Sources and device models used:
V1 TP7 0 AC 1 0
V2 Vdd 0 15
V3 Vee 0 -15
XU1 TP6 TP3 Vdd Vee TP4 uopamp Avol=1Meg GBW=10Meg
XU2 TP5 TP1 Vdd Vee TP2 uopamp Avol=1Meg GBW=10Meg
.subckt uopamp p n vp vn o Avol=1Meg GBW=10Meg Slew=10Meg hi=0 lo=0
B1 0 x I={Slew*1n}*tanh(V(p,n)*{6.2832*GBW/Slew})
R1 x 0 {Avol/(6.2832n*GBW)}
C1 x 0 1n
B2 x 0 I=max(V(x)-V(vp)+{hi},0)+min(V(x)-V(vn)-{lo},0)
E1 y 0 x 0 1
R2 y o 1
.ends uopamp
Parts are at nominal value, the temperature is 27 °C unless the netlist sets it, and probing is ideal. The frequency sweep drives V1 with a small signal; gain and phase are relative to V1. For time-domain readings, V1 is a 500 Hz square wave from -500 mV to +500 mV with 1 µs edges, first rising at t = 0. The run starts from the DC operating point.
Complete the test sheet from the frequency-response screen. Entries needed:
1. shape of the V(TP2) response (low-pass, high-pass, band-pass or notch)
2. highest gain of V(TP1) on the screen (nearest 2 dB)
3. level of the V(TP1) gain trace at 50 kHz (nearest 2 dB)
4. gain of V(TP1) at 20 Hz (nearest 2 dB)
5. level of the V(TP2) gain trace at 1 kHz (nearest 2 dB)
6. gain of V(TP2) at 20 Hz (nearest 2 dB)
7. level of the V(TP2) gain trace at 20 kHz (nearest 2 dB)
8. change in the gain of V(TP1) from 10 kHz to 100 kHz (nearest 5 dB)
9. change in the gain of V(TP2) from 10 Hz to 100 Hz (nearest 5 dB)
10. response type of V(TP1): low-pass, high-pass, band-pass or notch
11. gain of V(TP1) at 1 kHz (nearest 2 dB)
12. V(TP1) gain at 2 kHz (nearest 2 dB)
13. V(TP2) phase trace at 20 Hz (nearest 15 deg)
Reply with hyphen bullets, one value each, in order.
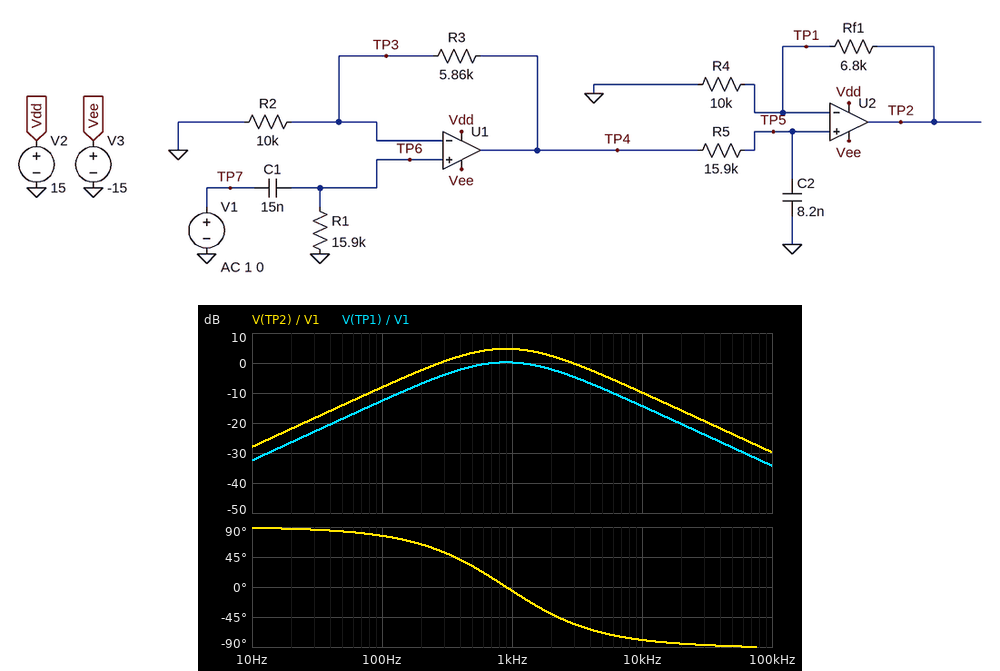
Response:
- band-pass
- 0 dB
- -28 dB
- -26 dB
- 4 dB
- -22 dB
- -16 dB
- -20 dB
- 20 dB
- band-pass
- 0 dB
- -2 dB
- 90 deg
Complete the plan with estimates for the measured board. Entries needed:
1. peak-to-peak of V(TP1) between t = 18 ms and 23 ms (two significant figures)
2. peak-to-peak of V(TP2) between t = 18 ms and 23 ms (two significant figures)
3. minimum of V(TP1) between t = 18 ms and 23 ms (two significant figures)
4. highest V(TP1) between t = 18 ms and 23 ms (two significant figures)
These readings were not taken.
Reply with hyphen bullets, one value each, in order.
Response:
- 1.5 V
- 2.5 V
- -740 mV
- 740 mV
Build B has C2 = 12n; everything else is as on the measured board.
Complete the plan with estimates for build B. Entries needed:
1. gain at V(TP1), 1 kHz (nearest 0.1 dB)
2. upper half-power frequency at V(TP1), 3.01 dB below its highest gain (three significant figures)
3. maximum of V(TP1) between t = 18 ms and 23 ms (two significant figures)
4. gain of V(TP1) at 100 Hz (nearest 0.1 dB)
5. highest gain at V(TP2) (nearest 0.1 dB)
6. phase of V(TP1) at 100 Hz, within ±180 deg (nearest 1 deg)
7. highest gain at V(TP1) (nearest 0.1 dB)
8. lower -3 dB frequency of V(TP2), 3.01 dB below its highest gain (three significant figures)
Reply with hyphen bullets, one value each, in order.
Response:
- -1.5 dB
- 1.81 kHz
- 620 mV
- -12.6 dB
- 3.4 dB
- 75 deg
- -1.1 dB
- 308 Hz
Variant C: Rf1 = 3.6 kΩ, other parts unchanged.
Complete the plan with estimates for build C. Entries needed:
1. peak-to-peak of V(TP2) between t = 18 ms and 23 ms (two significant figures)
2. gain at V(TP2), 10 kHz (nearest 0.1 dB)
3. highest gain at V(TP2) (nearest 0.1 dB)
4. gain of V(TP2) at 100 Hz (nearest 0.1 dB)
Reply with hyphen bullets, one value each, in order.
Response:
- 2.0 V
- -11.7 dB
- 2.9 dB
- -9.9 dB
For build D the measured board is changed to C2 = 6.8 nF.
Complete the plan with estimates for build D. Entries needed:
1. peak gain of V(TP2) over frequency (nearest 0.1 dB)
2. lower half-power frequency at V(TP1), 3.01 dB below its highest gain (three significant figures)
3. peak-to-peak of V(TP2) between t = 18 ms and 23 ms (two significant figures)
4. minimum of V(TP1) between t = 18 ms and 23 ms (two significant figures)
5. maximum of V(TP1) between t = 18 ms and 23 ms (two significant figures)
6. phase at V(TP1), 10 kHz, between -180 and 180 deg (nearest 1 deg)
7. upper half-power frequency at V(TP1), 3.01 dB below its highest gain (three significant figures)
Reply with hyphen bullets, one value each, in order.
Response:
- 5.3 dB
- 389 Hz
- 2.7 V
- -800 mV
- 800 mV
- -78 deg
- 2.53 kHz
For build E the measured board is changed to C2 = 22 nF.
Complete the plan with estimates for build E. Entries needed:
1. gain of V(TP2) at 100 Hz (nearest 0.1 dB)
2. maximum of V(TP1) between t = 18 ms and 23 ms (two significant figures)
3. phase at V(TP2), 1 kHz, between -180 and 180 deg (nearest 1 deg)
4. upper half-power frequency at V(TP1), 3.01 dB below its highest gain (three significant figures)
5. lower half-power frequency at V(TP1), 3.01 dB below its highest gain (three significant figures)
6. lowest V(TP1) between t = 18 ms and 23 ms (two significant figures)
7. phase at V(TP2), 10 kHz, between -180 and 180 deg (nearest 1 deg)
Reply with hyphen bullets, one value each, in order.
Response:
- -8.3 dB
- 410 mV
- -32 deg
- 1.35 kHz
- 225 Hz
- -410 mV
- -84 deg
